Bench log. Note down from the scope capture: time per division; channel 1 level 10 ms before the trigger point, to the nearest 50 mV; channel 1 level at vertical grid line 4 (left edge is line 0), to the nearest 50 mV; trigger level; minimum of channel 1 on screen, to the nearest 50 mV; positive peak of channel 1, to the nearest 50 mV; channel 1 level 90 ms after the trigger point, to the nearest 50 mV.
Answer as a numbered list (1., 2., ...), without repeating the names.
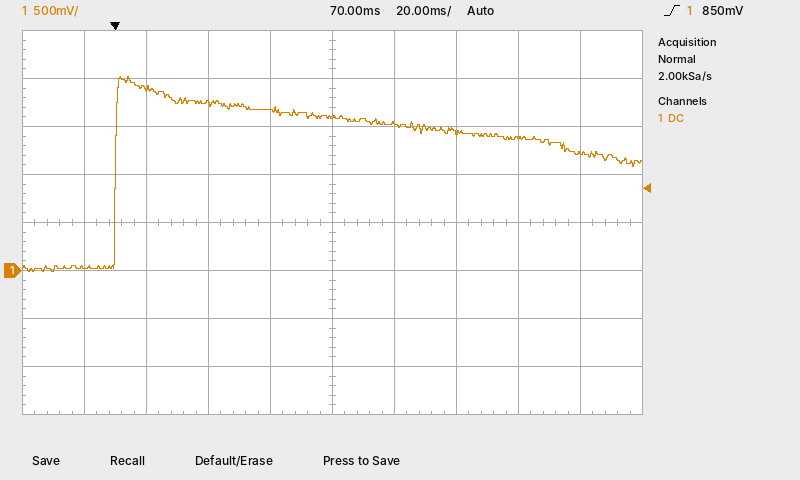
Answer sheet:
1. 20 ms
2. 50 mV
3. 1.65 V
4. 850 mV
5. 0 mV
6. 2.00 V
7. 1.55 V
